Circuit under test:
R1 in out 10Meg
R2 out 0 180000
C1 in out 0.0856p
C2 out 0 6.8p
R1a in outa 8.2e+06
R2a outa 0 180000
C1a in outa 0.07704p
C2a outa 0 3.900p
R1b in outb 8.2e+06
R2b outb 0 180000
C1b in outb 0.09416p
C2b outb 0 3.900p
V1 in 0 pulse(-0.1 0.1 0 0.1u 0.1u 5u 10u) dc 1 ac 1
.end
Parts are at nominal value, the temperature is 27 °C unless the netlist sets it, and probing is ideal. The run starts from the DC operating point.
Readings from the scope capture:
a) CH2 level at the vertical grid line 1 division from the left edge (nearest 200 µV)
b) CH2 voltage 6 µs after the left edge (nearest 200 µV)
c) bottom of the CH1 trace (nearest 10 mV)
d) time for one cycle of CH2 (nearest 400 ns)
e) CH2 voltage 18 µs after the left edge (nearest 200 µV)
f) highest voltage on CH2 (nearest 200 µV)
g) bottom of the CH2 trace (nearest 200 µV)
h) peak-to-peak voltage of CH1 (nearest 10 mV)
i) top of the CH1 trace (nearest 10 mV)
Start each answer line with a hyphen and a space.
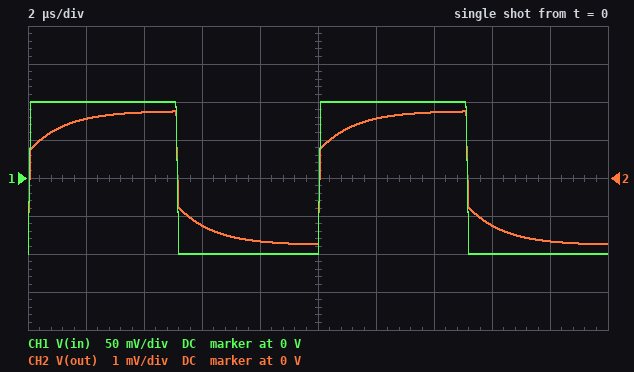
- 1.6 mV
- -1.2 mV
- -100 mV
- 10.0 µs
- -1.6 mV
- 1.8 mV
- -1.8 mV
- 200 mV
- 100 mV
